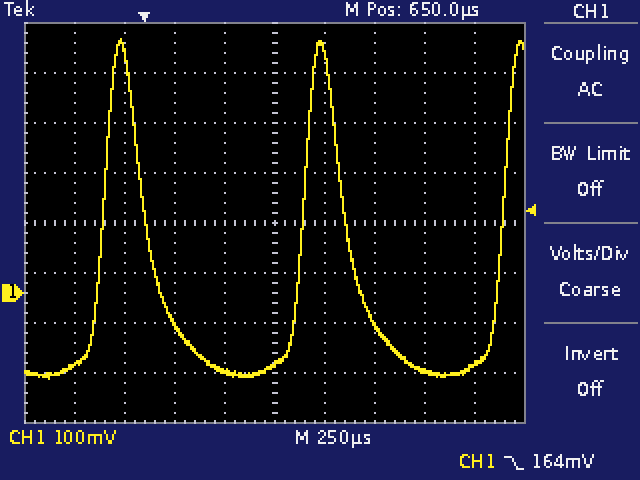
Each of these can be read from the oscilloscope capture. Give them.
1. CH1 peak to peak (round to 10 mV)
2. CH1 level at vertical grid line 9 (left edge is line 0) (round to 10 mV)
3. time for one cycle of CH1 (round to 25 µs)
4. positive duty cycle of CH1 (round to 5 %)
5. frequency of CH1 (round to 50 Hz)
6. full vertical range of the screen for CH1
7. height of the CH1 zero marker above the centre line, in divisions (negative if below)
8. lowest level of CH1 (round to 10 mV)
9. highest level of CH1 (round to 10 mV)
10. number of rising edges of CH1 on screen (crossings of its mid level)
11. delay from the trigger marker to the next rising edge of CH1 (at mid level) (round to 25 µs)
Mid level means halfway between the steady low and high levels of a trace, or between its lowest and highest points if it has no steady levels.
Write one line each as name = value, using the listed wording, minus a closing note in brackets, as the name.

CH1 peak to peak = 680 mV
CH1 level at vertical grid line 9 (left edge is line 0) = -140 mV
time for one cycle of CH1 = 1.000 ms
positive duty cycle of CH1 = 20 %
frequency of CH1 = 1.00 kHz
full vertical range of the screen for CH1 = 800 mV
height of the CH1 zero marker above the centre line, in divisions = -1.4 div
lowest level of CH1 = -170 mV
highest level of CH1 = 510 mV
number of rising edges of CH1 on screen = 3
delay from the trigger marker to the next rising edge of CH1 (at mid level) = 800 µs
